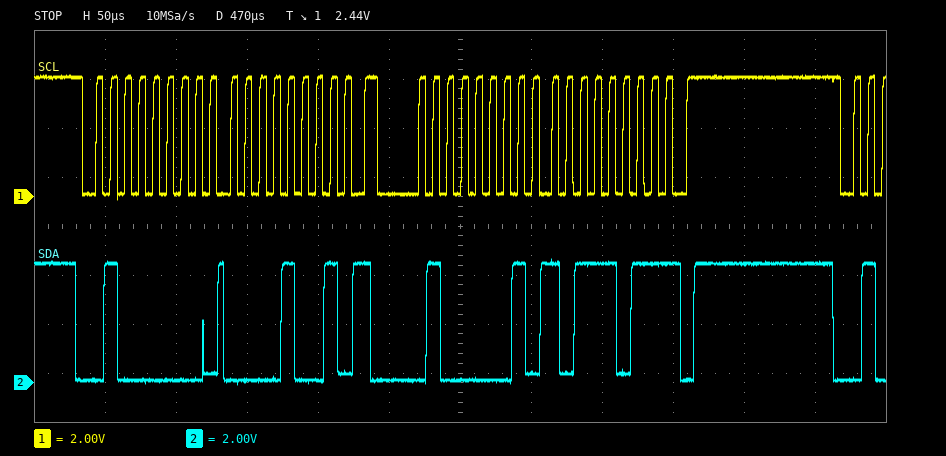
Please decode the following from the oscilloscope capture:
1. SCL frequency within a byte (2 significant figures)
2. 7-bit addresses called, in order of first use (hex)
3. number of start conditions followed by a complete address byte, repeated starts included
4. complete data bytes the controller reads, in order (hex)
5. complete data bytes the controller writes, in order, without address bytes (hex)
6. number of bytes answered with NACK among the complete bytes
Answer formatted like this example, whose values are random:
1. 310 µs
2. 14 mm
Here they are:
1. 100 kHz
2. 0x20
3. 2
4. BB
5. 09
6. 1
